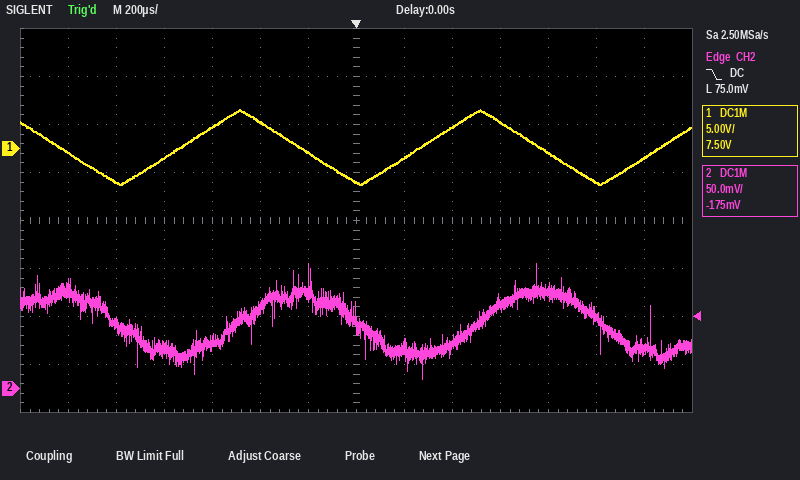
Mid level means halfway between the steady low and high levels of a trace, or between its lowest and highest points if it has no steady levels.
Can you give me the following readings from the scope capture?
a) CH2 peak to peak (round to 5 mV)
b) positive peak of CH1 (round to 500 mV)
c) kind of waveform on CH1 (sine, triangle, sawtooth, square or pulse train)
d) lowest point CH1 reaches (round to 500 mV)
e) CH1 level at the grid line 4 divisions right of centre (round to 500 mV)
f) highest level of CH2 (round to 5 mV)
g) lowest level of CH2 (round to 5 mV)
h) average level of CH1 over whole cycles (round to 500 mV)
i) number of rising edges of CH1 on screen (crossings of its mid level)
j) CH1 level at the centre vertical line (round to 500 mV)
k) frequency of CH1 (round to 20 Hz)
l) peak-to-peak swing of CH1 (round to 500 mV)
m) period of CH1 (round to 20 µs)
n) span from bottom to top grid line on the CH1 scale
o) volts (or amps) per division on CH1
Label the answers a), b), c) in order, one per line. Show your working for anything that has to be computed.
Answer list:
a) 130 mV − (10 mV) = 120 mV
b) 4.0 V
c) triangle
d) -4.0 V
e) -500 mV
f) 130 mV
g) 10 mV
h) (4.0 V + (-4.0 V)) / 2 ≈ 0.0 V
i) 3
j) -3.5 V
k) 1 / 1.00 ms ≈ 1.00 kHz
l) 4.0 V − (-4.0 V) = 8.0 V
m) 1.00 ms
n) 40 V
o) 5 V
